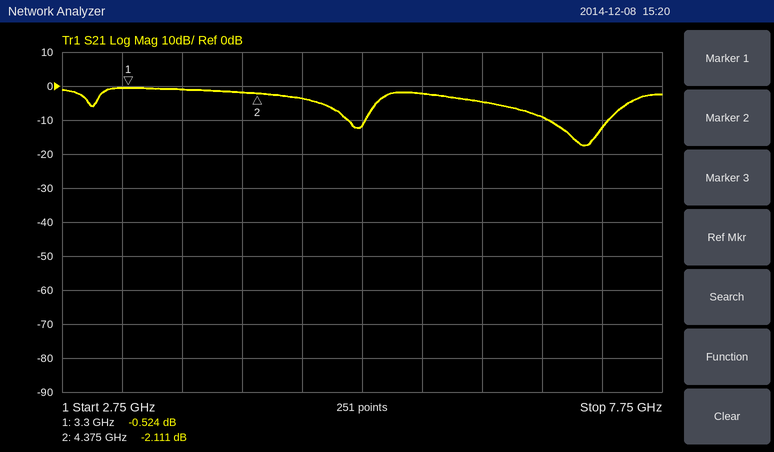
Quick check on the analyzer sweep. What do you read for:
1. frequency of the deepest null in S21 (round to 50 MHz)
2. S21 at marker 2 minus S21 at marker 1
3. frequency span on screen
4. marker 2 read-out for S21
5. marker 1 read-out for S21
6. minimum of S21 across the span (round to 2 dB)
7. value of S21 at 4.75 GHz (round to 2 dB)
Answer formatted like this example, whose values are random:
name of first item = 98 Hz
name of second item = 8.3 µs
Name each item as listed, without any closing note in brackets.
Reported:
frequency of the deepest null in S21 = 7.10 GHz
S21 at marker 2 minus S21 at marker 1 = -1.587 dB
frequency span on screen = 5 GHz
marker 2 read-out for S21 = -2.111 dB
marker 1 read-out for S21 = -0.524 dB
minimum of S21 across the span = -18 dB
value of S21 at 4.75 GHz = -4 dB
